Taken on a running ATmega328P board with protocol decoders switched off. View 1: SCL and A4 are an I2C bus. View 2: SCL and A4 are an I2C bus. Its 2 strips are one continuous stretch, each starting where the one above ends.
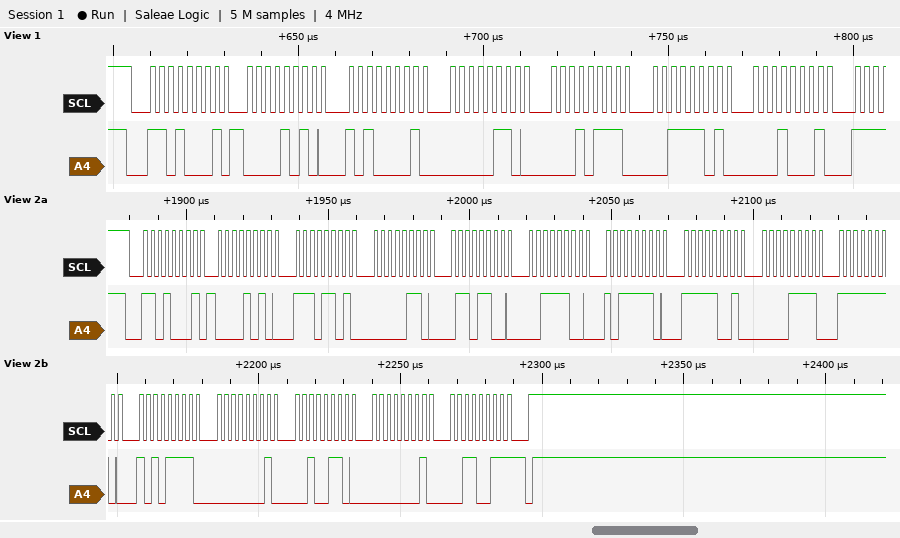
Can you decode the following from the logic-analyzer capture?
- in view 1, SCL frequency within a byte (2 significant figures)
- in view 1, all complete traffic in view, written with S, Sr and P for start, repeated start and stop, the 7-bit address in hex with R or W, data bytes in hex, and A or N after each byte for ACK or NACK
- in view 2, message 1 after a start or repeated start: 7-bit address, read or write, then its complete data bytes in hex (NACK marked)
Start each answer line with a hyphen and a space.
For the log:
- 400 kHz
- S 68R A 0A A A1 A 06 A 17 A 3D A 11 A
- 0x68 read: 0A ED 06 6C 3C BE F9 0F FE AF 01 26 01 33 NACK
